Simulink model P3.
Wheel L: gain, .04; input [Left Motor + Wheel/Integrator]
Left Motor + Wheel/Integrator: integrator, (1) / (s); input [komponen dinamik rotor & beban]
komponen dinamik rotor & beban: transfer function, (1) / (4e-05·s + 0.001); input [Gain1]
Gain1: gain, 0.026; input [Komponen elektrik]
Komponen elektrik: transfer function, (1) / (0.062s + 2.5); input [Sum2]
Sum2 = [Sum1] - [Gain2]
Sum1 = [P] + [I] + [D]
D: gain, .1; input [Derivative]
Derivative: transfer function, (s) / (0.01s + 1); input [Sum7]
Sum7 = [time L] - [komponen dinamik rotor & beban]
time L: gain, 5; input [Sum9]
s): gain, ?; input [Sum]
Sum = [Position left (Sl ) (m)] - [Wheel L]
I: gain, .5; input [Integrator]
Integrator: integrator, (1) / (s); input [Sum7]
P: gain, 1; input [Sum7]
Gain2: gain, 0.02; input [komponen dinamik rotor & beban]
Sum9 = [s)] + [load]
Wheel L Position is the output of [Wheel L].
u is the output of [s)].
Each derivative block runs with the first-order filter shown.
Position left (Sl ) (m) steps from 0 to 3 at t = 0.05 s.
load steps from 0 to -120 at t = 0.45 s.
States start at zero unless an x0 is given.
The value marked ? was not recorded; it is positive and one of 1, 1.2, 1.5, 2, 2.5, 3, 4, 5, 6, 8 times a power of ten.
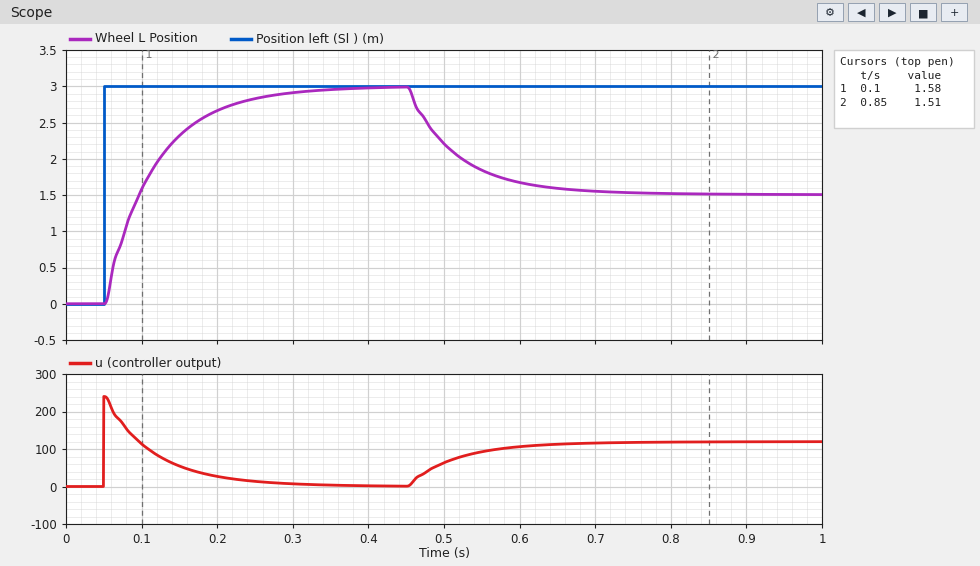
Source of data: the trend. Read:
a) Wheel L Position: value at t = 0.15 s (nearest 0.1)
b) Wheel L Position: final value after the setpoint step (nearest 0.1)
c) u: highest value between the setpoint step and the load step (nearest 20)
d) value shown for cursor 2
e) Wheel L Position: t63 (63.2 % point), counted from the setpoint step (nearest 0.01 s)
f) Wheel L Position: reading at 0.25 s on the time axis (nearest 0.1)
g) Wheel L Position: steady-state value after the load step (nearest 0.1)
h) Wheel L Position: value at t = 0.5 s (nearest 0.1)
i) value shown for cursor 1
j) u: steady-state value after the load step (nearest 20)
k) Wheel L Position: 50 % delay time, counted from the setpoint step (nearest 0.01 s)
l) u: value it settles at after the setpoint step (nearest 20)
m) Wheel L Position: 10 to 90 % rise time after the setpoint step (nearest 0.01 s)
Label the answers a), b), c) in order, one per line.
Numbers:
a) 2.3
b) 3.0
c) 240
d) 1.51
e) 0.07 s
f) 2.8
g) 1.5
h) 2.2
i) 1.58
j) 120
k) 0.05 s
l) 0
m) 0.15 s
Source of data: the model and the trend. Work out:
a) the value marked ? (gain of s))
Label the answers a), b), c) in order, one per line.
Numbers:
a) 80
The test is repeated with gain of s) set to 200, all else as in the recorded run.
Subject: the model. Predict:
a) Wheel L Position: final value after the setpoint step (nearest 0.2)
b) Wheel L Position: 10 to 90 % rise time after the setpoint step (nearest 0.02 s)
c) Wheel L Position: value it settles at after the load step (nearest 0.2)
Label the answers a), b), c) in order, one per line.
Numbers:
a) 3.0
b) 0.06 s
c) 2.4
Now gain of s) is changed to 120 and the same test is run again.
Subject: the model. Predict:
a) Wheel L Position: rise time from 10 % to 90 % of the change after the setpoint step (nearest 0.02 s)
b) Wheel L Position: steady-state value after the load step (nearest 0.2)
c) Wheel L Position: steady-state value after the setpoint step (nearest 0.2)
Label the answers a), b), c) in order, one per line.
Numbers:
a) 0.10 s
b) 2.0
c) 3.0
